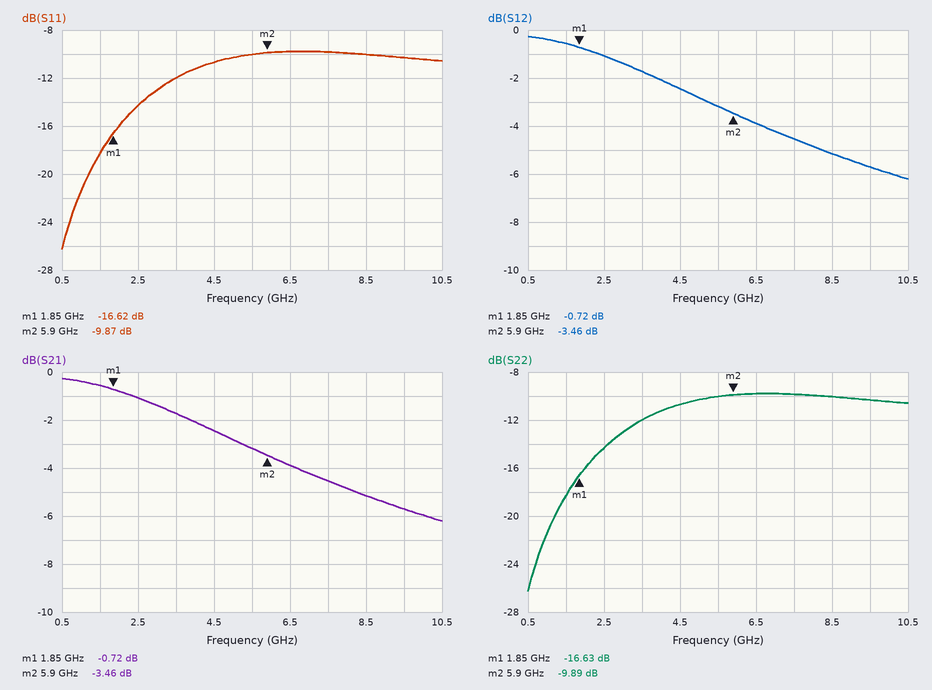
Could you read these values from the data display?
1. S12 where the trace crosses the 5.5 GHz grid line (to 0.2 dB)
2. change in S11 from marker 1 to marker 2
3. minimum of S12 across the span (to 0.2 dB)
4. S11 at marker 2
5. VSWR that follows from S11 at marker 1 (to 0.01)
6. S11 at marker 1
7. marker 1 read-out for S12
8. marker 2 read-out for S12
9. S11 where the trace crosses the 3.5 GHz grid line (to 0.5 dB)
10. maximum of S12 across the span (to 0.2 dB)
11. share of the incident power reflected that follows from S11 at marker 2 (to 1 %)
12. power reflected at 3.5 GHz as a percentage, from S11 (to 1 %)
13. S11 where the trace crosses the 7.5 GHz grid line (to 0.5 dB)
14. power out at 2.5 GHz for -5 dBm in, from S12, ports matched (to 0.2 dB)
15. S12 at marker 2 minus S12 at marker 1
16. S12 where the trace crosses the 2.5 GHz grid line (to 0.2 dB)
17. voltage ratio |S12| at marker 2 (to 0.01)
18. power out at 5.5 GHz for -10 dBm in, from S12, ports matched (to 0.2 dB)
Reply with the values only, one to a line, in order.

-3.2 dB
6.75 dB
-6.2 dB
-9.87 dB
1.35
-16.62 dB
-0.72 dB
-3.46 dB
-12.0 dB
-0.2 dB
10 %
6 %
-10.0 dB
-6.0 dBm
-2.74 dB
-1.0 dB
0.67
-13.2 dBm
